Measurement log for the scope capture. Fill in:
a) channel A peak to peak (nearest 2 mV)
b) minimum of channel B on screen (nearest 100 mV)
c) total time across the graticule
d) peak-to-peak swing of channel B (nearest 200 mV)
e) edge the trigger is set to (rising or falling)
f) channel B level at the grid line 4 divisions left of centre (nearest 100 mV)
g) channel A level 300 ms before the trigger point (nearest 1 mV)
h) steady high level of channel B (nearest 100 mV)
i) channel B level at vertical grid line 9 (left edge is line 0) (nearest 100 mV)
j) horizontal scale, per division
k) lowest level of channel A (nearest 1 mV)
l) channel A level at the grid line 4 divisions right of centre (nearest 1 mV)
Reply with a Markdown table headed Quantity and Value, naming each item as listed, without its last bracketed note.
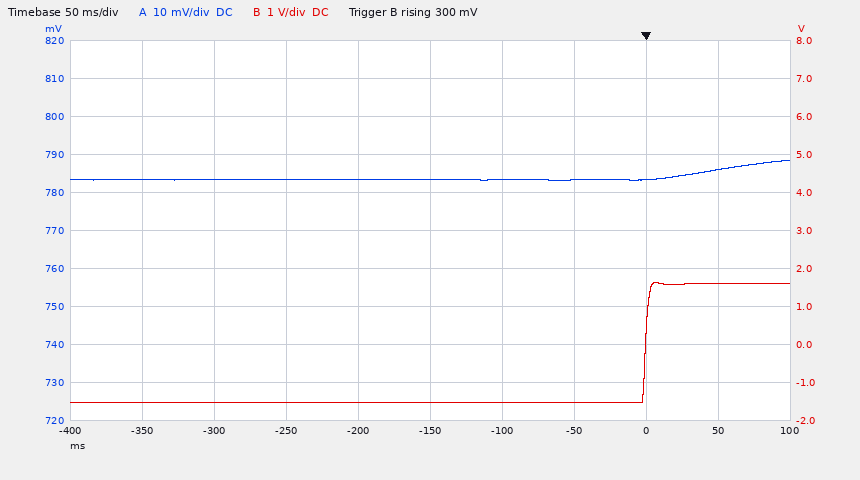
| Quantity | Value |
|---|---|
| channel A peak to peak | 6 mV |
| minimum of channel B on screen | -1.5 V |
| total time across the graticule | 500 ms |
| peak-to-peak swing of channel B | 3.2 V |
| edge the trigger is set to | rising |
| channel B level at the grid line 4 divisions left of centre | -1.5 V |
| channel A level 300 ms before the trigger point | 783 mV |
| steady high level of channel B | 1.6 V |
| channel B level at vertical grid line 9 (left edge is line 0) | 1.6 V |
| horizontal scale, per division | 50 ms |
| lowest level of channel A | 783 mV |
| channel A level at the grid line 4 divisions right of centre | 786 mV |
